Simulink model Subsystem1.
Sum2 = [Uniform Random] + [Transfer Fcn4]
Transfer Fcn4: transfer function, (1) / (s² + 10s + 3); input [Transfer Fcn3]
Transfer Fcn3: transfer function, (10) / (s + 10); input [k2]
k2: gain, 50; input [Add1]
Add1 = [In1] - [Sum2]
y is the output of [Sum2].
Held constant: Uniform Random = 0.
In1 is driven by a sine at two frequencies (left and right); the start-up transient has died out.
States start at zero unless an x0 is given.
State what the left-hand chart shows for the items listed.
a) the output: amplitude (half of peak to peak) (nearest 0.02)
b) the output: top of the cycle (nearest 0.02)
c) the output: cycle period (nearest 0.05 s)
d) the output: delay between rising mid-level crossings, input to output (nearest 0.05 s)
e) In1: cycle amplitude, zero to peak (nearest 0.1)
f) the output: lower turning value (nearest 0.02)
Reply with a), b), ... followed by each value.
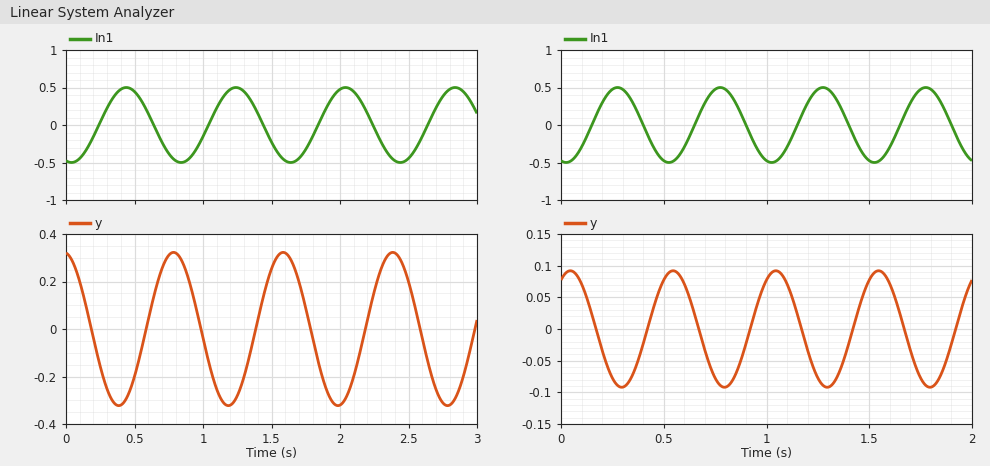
a) 0.32
b) 0.32
c) 0.80 s
d) 0.35 s
e) 0.5
f) -0.32
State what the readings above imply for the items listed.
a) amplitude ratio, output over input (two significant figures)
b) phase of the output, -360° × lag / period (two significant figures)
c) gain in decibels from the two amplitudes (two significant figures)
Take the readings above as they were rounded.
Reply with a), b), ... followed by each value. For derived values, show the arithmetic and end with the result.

a) 0.32 / 0.5 = 0.64
b) -360 × 0.35 / 0.8 = -160°
c) 20 log10(0.32 / 0.5) = -3.9 dB
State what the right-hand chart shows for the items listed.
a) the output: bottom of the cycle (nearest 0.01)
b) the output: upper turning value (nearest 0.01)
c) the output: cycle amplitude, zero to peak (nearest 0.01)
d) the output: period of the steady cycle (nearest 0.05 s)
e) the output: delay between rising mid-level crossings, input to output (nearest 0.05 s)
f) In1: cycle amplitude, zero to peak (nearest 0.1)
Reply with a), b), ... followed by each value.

a) -0.09
b) 0.09
c) 0.09
d) 0.50 s
e) 0.25 s
f) 0.5
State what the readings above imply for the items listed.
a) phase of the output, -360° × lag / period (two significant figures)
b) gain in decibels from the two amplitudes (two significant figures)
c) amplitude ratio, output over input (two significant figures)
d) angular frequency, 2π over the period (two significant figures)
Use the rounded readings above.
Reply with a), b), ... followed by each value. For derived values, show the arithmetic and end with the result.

a) -360 × 0.25 / 0.5 = -180°
b) 20 log10(0.09 / 0.5) = -15 dB
c) 0.09 / 0.5 = 0.18
d) 2π / 0.5 = 13 rad/s
